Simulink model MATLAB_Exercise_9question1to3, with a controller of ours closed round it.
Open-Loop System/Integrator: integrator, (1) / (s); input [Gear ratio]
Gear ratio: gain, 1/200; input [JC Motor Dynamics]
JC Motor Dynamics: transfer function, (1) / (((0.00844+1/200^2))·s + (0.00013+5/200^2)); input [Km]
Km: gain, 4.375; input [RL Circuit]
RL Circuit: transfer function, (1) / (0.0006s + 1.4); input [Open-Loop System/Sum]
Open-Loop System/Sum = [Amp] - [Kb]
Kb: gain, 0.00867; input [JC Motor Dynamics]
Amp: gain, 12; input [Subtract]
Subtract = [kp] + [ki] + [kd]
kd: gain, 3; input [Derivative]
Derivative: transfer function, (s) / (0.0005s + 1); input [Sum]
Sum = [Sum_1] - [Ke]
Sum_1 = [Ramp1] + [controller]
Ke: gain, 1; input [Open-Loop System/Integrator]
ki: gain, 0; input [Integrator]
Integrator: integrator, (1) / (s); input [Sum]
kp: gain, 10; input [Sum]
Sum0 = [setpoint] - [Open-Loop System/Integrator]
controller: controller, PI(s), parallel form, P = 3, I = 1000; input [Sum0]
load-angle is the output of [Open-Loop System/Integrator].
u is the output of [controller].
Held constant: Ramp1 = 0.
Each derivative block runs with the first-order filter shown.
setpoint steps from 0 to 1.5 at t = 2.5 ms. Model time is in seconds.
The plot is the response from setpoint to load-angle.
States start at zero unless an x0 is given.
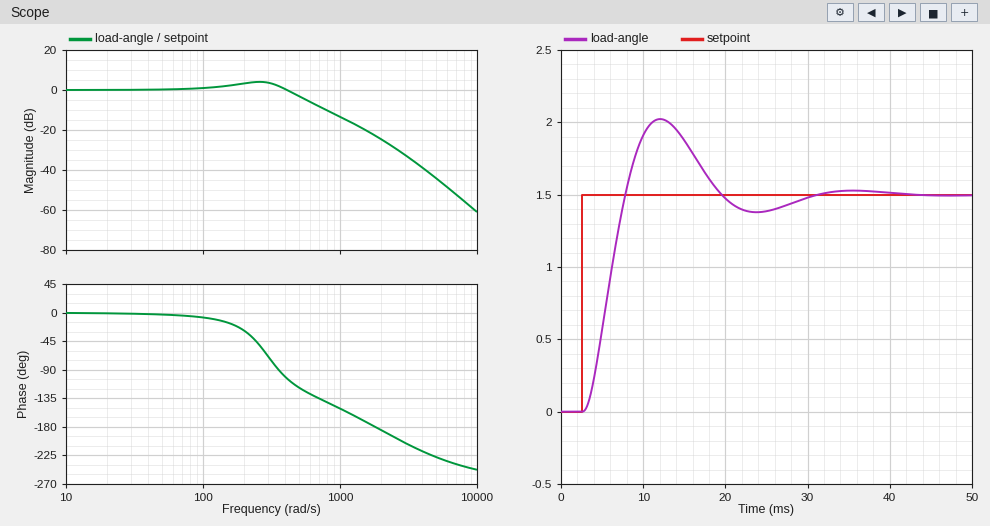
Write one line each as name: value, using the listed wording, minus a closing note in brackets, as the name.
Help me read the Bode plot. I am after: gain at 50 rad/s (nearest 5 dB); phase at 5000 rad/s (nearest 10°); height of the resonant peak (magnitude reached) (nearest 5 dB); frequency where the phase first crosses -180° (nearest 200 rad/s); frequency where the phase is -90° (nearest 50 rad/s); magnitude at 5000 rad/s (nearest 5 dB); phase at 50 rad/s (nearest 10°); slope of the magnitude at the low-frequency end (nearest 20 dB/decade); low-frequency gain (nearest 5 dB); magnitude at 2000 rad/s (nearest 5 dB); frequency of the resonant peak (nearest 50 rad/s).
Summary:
gain at 50 rad/s: 0 dB
phase at 5000 rad/s: -230°
height of the resonant peak (magnitude reached): 5 dB
frequency where the phase first crosses -180°: 1800 rad/s
frequency where the phase is -90°: 350 rad/s
magnitude at 5000 rad/s: -45 dB
phase at 50 rad/s: 0°
slope of the magnitude at the low-frequency end: 0 dB/decade
low-frequency gain: 0 dB
magnitude at 2000 rad/s: -25 dB
frequency of the resonant peak: 250 rad/s
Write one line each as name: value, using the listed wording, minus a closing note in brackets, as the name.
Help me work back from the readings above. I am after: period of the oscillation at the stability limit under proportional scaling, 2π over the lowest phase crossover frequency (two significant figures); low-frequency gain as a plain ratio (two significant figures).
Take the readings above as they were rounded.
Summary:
period of the oscillation at the stability limit under proportional scaling, 2π over the lowest phase crossover frequency: 0.0035 s
low-frequency gain as a plain ratio: 1.0
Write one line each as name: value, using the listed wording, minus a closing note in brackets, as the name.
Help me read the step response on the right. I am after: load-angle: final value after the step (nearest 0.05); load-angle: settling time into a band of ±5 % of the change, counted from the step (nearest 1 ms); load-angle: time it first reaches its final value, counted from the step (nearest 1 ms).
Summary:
load-angle: final value after the step: 1.50
load-angle: settling time into a band of ±5 % of the change, counted from the step: 25 ms
load-angle: time it first reaches its final value, counted from the step: 5 ms
